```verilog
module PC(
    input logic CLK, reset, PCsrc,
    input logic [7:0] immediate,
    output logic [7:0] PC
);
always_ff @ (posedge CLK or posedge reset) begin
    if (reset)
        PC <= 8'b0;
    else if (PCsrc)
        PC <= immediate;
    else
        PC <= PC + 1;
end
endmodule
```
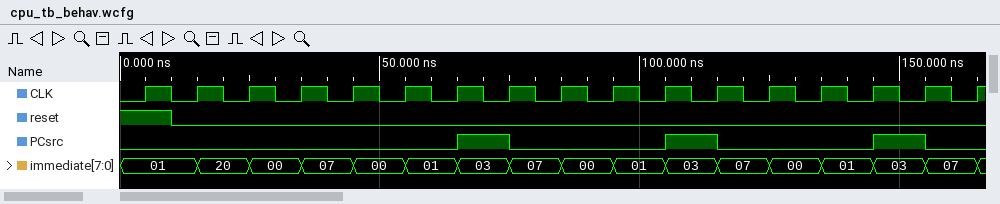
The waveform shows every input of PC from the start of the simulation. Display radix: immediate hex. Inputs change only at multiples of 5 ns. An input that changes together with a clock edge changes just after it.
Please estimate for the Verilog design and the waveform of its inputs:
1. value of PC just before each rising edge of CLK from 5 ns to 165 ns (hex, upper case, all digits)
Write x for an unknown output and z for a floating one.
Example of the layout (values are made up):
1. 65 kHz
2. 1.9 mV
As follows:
1. 00, 00, 01, 02, 03, 04, 05, 06, 03, 04, 05, 06, 03, 04, 05, 06, 03
